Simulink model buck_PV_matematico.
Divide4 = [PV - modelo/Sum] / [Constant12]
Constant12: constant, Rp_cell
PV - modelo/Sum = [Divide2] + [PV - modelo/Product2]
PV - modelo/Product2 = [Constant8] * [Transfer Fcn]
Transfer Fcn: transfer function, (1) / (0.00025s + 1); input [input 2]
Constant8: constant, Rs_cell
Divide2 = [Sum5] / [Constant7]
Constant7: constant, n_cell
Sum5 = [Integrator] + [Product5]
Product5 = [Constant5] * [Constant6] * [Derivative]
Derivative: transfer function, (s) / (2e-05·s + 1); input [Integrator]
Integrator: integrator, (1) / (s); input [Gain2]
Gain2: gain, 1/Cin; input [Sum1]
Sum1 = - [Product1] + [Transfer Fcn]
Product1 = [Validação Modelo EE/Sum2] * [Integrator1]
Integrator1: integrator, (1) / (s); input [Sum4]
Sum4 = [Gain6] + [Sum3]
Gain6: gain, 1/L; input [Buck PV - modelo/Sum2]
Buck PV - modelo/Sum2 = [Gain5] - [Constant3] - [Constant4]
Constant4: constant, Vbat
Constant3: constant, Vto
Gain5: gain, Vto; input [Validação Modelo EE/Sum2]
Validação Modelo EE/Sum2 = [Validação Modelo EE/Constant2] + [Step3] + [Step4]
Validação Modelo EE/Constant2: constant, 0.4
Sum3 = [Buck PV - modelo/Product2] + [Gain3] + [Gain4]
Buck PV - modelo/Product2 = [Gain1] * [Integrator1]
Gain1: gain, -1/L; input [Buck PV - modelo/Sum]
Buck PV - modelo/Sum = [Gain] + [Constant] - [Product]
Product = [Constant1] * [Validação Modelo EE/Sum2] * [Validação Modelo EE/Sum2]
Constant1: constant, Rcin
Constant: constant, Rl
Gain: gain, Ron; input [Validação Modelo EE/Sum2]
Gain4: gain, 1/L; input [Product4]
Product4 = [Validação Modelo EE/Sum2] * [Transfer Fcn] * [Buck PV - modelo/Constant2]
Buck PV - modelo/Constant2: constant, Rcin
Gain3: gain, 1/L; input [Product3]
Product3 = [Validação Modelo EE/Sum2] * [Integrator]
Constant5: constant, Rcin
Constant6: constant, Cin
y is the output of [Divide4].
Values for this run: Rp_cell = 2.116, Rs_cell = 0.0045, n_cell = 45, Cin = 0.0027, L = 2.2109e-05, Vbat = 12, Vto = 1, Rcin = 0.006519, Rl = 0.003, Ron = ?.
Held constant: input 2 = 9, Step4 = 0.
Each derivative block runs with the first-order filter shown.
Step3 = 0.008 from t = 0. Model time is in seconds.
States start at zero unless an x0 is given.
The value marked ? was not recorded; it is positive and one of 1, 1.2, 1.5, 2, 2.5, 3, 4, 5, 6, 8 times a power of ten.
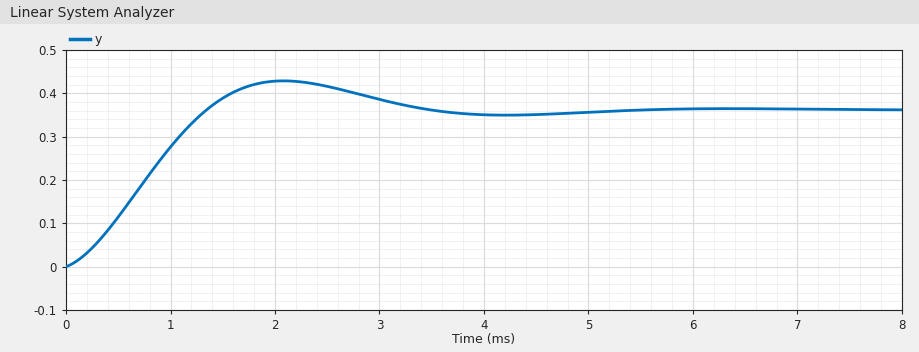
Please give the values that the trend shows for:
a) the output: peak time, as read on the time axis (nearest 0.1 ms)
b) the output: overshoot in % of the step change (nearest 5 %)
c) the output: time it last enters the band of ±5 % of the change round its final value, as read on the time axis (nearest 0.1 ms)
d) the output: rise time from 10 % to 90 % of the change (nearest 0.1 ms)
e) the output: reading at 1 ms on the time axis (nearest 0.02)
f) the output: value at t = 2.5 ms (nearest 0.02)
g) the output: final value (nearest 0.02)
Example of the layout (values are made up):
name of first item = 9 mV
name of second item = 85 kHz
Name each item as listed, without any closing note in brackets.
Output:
the output: peak time, as read on the time axis = 2.1 ms
the output: overshoot in % of the step change = 20 %
the output: time it last enters the band of ±5 % of the change round its final value, as read on the time axis = 3.1 ms
the output: rise time from 10 % to 90 % of the change = 1.0 ms
the output: reading at 1 ms on the time axis = 0.28
the output: value at t = 2.5 ms = 0.42
the output: final value = 0.36
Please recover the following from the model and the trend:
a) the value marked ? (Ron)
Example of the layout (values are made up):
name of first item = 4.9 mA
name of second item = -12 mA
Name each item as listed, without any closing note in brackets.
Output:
the value marked ? = 0.08
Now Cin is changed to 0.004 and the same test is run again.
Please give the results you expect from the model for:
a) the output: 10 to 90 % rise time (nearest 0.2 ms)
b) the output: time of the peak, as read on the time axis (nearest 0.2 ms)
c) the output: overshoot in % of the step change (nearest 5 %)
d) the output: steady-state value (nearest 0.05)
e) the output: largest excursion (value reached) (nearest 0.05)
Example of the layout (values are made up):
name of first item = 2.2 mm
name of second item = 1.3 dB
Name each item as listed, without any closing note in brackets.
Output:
the output: 10 to 90 % rise time = 1.4 ms
the output: time of the peak, as read on the time axis = 2.8 ms
the output: overshoot in % of the step change = 10 %
the output: steady-state value = 0.35
the output: largest excursion (value reached) = 0.40
